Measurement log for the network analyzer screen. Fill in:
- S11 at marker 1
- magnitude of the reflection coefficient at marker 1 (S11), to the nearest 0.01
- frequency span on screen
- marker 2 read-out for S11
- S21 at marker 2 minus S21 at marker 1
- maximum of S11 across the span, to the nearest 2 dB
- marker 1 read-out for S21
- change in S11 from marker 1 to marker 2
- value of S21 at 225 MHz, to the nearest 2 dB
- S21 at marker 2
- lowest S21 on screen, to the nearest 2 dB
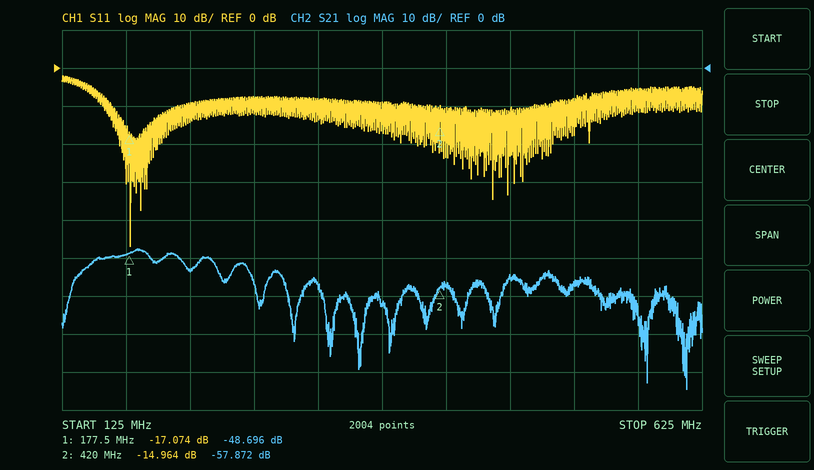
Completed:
-17.074 dB
0.14
500 MHz
-14.964 dB
-9.176 dB
-2 dB
-48.696 dB
2.110 dB
-54 dB
-57.872 dB
-84 dB
